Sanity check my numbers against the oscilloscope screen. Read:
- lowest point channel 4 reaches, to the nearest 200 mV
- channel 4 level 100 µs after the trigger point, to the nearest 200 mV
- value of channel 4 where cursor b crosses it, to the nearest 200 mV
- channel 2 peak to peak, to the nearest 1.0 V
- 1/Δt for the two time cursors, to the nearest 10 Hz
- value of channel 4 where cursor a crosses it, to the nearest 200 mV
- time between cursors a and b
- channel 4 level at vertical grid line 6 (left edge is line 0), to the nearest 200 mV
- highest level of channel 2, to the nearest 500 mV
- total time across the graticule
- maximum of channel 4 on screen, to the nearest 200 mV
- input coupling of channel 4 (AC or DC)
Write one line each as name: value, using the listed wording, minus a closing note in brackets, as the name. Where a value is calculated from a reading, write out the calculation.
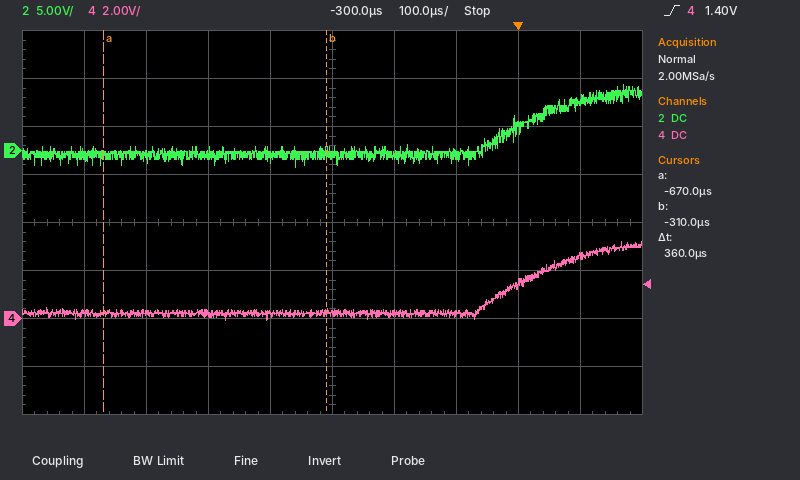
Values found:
lowest point channel 4 reaches, to the nearest 200 mV: 0.0 V
channel 4 level 100 µs after the trigger point, to the nearest 200 mV: 2.6 V
value of channel 4 where cursor b crosses it, to the nearest 200 mV: 200 mV
channel 2 peak to peak, to the nearest 1.0 V: 9.0 V
1/Δt for the two time cursors, to the nearest 10 Hz: 1 / 360 µs ≈ 2.78 kHz
value of channel 4 where cursor a crosses it, to the nearest 200 mV: 200 mV
time between cursors a and b: 360 µs
channel 4 level at vertical grid line 6 (left edge is line 0), to the nearest 200 mV: 200 mV
highest level of channel 2, to the nearest 500 mV: 7.0 V
total time across the graticule: 1 ms
maximum of channel 4 on screen, to the nearest 200 mV: 3.2 V
input coupling of channel 4: DC
